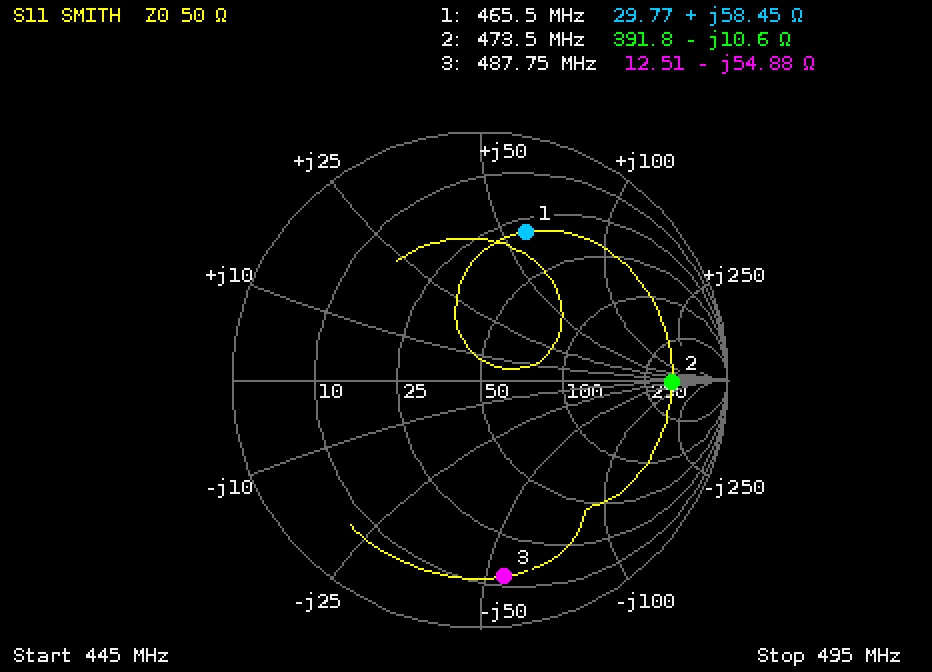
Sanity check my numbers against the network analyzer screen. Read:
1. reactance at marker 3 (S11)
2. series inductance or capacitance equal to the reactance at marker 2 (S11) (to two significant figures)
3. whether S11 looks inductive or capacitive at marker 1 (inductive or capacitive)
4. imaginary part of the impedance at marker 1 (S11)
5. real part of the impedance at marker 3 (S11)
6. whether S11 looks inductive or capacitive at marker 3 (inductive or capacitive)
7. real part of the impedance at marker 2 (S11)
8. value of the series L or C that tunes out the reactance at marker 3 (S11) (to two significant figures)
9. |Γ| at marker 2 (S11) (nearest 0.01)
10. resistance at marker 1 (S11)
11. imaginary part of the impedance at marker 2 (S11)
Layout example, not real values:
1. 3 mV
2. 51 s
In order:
1. -54.88 Ω
2. 32 pF
3. inductive
4. +58.45 Ω
5. 12.51 Ω
6. capacitive
7. 391.8 Ω
8. 18 nH
9. 0.77
10. 29.77 Ω
11. -10.6 Ω
